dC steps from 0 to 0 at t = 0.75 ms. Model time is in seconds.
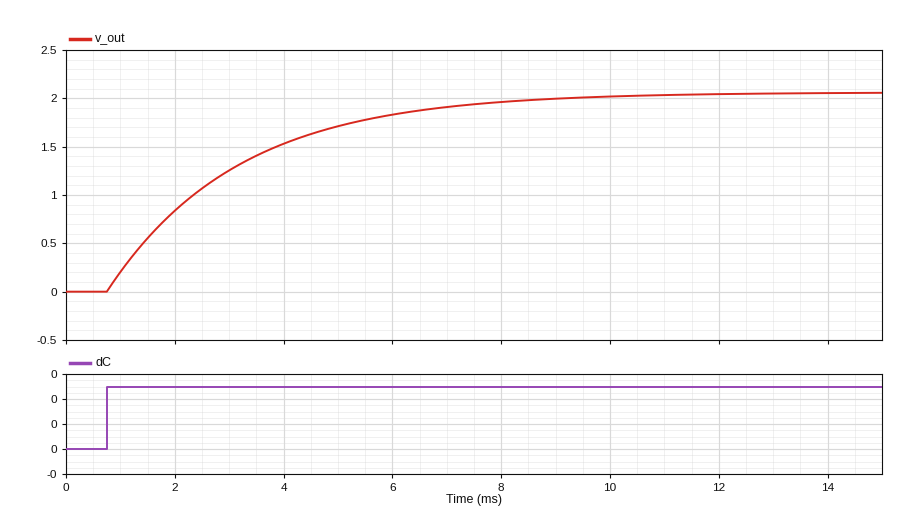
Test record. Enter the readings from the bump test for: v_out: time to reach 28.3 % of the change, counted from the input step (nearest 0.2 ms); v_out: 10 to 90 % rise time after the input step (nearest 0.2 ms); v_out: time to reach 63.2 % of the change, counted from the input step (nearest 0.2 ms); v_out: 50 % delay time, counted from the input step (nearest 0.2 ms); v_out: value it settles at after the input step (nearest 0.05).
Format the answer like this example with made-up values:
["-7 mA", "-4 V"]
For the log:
["0.8 ms", "5.2 ms", "2.4 ms", "1.6 ms", "2.05"]
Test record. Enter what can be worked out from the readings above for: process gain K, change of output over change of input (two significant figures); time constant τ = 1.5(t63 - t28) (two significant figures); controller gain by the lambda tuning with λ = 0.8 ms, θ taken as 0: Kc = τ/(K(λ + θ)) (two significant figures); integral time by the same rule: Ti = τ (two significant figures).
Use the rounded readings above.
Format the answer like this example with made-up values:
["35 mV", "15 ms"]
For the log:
["41000000000000", "2.4 ms", "0.000000000000073", "2.4 ms"]
